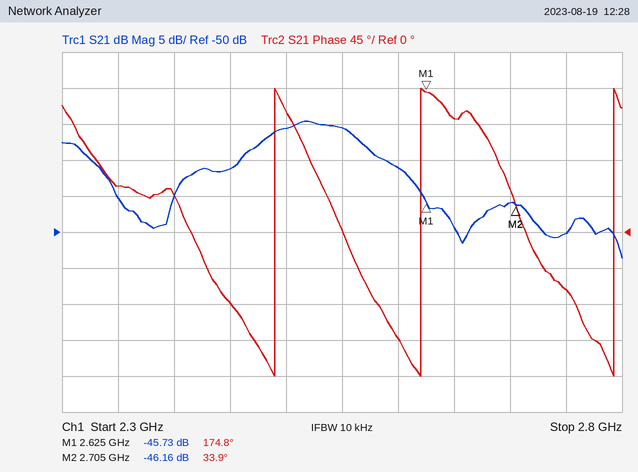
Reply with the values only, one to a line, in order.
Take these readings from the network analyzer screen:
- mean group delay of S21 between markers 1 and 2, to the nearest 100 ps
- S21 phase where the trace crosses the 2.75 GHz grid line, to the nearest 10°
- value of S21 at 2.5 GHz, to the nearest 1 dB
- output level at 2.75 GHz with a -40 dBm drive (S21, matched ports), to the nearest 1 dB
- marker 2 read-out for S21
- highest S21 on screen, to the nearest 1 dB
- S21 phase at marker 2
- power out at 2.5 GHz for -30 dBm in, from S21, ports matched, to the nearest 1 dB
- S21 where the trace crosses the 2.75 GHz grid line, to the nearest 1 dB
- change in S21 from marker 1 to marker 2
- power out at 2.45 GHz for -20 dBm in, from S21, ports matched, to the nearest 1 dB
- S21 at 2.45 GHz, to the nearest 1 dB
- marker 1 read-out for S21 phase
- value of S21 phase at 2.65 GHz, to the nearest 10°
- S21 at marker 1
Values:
4.9 ns
-70°
-36 dB
-90 dBm
-46.16 dB
-35 dB
33.9°
-66 dBm
-50 dB
-0.43 dB
-61 dBm
-41 dB
174.8°
140°
-45.73 dB
